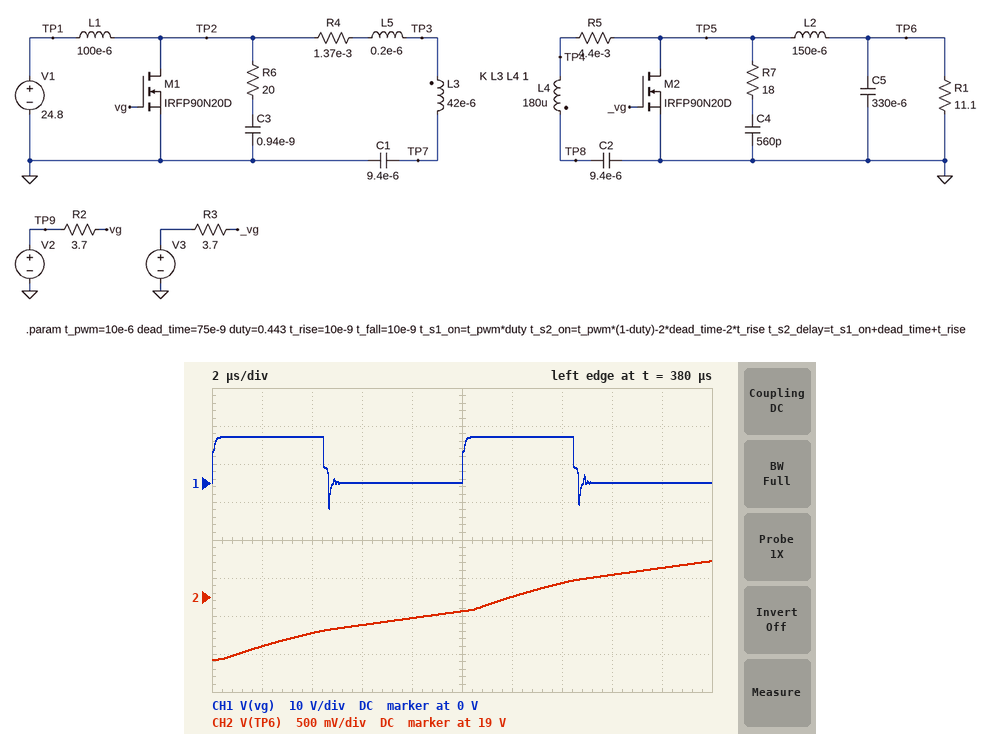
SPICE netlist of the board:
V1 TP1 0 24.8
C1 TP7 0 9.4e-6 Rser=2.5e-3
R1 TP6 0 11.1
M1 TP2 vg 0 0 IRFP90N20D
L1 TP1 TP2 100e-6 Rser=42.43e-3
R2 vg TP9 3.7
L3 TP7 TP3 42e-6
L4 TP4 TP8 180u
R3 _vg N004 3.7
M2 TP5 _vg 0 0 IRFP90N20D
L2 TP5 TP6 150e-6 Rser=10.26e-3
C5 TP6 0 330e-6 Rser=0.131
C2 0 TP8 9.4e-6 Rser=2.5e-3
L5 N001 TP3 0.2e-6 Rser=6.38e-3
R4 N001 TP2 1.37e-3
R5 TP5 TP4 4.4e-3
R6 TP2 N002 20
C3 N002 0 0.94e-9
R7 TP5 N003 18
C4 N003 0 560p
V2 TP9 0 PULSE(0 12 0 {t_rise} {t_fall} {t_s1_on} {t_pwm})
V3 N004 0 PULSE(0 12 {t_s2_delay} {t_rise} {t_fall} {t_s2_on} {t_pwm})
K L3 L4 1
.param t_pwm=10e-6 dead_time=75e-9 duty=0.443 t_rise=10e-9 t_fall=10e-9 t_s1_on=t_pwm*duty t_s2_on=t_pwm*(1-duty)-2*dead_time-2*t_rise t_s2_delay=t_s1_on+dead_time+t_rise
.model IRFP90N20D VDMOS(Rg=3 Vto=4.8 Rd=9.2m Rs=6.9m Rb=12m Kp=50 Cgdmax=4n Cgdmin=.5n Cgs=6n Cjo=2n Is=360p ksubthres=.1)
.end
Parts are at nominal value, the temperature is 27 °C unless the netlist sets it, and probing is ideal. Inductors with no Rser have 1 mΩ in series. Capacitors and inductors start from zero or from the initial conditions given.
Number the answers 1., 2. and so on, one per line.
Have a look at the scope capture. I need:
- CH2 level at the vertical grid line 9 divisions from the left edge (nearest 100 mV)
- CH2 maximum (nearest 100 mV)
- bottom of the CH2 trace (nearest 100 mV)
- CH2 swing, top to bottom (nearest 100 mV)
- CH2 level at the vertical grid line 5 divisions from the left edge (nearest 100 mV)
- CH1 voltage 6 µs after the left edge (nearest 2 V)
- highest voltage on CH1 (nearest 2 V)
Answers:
1. 19.4 V
2. 19.5 V
3. 18.2 V
4. 1.3 V
5. 18.8 V
6. 0 V
7. 12 V
